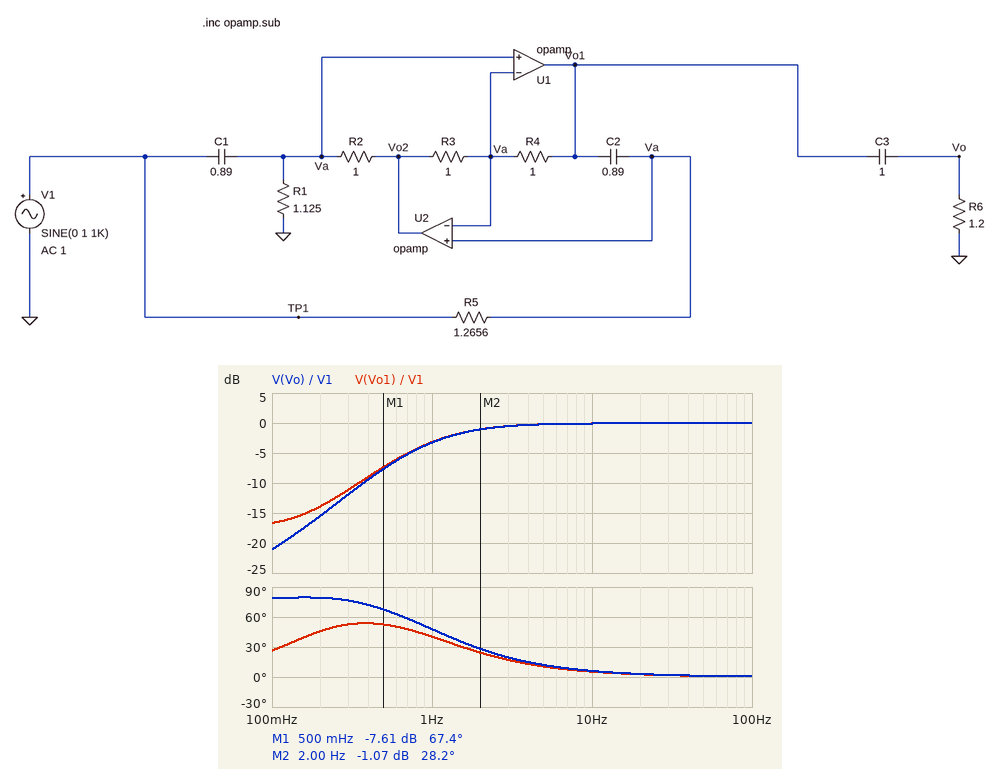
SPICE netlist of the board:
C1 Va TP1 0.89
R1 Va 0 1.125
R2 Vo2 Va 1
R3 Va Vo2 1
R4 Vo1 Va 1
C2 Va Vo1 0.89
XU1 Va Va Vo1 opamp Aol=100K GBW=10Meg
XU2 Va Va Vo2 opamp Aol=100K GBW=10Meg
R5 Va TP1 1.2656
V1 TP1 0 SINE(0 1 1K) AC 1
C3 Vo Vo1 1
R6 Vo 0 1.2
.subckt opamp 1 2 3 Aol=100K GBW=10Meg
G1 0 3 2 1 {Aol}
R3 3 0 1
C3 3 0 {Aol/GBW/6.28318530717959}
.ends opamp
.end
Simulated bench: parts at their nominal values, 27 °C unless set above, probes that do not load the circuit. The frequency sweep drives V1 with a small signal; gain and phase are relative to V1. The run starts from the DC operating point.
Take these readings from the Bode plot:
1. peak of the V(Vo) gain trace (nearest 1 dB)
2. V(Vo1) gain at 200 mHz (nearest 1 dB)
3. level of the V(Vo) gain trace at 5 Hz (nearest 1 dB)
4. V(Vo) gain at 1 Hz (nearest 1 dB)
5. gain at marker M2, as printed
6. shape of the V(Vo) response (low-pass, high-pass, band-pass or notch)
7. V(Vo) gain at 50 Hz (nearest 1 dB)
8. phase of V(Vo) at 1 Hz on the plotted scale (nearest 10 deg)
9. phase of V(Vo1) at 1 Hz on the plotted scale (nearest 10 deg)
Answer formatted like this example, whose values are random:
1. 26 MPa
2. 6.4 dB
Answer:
1. 0 dB
2. -14 dB
3. 0 dB
4. -3 dB
5. -1.07 dB
6. high-pass
7. 0 dB
8. 50 deg
9. 40 deg
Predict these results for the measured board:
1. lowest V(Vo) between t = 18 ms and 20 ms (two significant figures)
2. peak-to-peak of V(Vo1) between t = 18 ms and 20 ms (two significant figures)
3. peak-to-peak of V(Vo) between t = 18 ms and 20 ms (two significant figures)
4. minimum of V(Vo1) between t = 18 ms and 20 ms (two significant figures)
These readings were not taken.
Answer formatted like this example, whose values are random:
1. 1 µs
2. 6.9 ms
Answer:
1. -1.0 V
2. 2.0 V
3. 2.0 V
4. -1.0 V
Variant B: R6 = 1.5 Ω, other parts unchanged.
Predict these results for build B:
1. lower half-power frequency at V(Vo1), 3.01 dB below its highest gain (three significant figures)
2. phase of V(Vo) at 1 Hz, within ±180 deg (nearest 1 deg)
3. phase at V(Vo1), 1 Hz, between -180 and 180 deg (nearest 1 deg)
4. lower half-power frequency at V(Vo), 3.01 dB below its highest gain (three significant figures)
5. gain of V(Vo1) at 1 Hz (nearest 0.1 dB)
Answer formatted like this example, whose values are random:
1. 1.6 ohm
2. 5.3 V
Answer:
1. 964 mHz
2. 45 deg
3. 39 deg
4. 976 mHz
5. -2.9 dB
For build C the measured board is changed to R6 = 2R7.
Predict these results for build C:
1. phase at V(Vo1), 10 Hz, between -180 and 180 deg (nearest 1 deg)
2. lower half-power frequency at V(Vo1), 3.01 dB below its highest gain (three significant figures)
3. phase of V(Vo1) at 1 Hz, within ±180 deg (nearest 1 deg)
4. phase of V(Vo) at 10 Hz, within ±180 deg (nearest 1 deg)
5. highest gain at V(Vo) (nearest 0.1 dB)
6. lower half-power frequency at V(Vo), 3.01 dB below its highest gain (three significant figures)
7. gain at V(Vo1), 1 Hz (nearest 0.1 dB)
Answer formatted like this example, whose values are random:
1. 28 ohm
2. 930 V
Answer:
1. 4 deg
2. 847 mHz
3. 36 deg
4. 5 deg
5. 0 dB
6. 851 mHz
7. -2.4 dB
